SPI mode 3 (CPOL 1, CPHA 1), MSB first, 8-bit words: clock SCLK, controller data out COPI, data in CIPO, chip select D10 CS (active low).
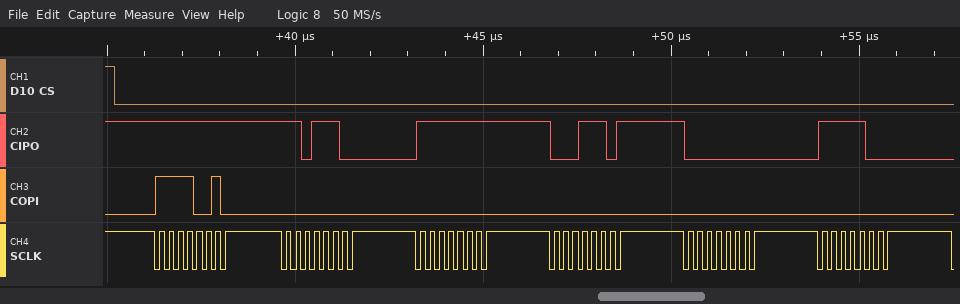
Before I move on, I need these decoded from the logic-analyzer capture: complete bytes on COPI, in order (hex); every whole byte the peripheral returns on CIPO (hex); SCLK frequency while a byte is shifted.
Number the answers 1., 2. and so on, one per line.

1. F2 00 00 00 00 00
2. FF DC FF 1D 00 F8
3. 4 MHz
